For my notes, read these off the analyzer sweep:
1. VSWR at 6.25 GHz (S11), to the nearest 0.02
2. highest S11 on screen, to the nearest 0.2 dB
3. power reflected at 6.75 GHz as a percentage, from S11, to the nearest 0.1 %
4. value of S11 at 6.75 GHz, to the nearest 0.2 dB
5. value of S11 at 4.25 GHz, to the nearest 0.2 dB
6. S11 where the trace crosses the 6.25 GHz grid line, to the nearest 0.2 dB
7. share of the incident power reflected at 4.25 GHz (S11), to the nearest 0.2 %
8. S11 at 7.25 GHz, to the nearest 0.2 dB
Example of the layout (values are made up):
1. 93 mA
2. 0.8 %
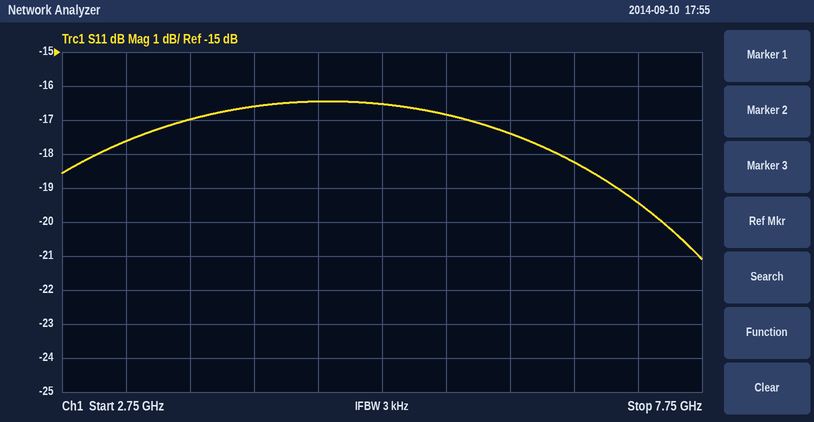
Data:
1. 1.32
2. -16.4 dB
3. 1.5 %
4. -18.2 dB
5. -16.6 dB
6. -17.4 dB
7. 2.2 %
8. -19.4 dB
